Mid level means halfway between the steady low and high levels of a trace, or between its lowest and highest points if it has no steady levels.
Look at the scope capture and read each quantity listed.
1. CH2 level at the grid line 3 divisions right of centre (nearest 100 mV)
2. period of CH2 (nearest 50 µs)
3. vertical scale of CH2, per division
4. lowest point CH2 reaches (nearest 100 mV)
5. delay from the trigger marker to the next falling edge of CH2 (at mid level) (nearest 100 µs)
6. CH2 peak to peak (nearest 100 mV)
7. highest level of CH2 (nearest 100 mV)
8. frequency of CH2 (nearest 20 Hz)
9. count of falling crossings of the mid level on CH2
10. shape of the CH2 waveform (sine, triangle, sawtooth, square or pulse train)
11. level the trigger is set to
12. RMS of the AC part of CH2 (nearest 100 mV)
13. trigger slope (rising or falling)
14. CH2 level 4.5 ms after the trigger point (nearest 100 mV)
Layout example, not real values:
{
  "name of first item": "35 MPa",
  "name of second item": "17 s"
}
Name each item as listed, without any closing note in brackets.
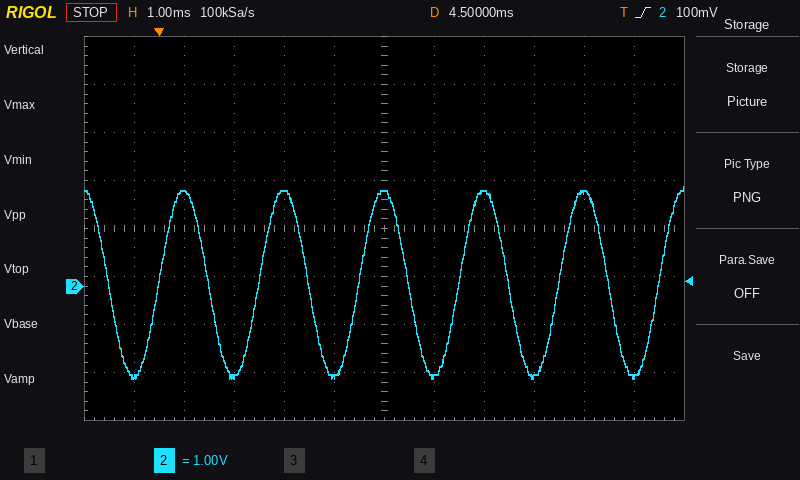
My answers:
{
  "CH2 level at the grid line 3 divisions right of centre": "-1.9 V",
  "period of CH2": "2.00 ms",
  "vertical scale of CH2, per division": "1 V",
  "lowest point CH2 reaches": "-1.9 V",
  "delay from the trigger marker to the next falling edge of CH2 (at mid level)": "1.0 ms",
  "CH2 peak to peak": "4.0 V",
  "highest level of CH2": "2.1 V",
  "frequency of CH2": "500 Hz",
  "count of falling crossings of the mid level on CH2": "6",
  "shape of the CH2 waveform": "sine",
  "level the trigger is set to": "100 mV",
  "RMS of the AC part of CH2": "1.4 V",
  "trigger slope": "rising",
  "CH2 level 4.5 ms after the trigger point": "2.0 V"
}
